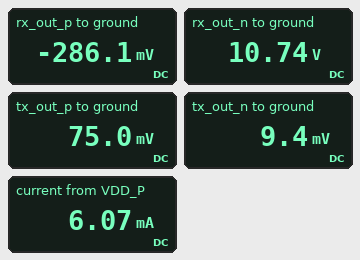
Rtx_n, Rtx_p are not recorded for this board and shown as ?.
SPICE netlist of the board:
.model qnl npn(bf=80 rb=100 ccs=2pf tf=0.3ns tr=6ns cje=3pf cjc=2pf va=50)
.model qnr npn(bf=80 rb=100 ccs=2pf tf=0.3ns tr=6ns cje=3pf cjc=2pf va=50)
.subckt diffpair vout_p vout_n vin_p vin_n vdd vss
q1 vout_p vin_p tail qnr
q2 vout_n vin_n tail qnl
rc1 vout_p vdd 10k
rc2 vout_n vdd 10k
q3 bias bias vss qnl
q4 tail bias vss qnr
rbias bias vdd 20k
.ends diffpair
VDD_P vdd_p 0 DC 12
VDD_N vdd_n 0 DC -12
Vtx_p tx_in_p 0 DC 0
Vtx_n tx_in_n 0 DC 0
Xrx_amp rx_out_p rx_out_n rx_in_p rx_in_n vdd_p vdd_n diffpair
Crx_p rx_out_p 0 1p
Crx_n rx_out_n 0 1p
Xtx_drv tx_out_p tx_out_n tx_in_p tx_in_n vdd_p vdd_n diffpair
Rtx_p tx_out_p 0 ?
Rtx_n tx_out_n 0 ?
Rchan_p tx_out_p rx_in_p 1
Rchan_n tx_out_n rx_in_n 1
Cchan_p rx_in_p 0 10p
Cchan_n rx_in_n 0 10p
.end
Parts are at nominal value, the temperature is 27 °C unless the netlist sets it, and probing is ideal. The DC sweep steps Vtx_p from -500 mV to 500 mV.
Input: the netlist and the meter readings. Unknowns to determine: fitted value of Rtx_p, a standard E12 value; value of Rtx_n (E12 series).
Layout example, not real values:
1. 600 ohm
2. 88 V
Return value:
1. 150 Ω
2. 18 Ω
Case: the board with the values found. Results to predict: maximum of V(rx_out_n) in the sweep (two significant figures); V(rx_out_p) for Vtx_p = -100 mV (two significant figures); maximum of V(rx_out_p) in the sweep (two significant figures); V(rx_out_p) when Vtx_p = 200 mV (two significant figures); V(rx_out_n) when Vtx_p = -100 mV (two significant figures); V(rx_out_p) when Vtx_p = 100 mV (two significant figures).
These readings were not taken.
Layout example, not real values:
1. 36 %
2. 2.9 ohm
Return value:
1. 12 V
2. -570 mV
3. 9.7 V
4. 9.6 V
5. 12 V
6. 9.2 V
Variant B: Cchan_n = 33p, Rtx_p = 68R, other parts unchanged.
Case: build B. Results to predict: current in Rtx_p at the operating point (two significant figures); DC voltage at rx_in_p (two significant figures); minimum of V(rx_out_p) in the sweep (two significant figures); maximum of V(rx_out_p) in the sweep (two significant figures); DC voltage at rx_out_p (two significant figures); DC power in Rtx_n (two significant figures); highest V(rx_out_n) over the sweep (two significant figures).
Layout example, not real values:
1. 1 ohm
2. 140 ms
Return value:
1. 510 µA
2. 35 mV
3. -590 mV
4. 8.6 V
5. 2.5 V
6. 4.8 µW
7. 11 V
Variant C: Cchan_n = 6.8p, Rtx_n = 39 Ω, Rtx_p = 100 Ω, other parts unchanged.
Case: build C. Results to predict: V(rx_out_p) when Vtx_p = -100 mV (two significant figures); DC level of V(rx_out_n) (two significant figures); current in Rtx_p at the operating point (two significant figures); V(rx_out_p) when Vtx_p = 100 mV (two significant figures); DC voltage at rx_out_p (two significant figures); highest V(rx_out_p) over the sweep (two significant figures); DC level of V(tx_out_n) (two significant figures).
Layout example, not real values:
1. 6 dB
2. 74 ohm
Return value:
1. -600 mV
2. 8.4 V
3. 510 µA
4. 10 V
5. 2.0 V
6. 11 V
7. 20 mV
